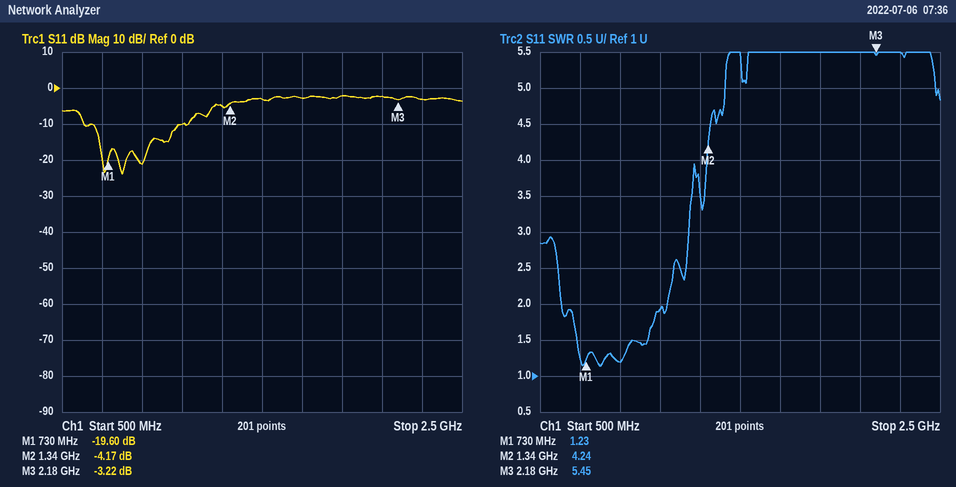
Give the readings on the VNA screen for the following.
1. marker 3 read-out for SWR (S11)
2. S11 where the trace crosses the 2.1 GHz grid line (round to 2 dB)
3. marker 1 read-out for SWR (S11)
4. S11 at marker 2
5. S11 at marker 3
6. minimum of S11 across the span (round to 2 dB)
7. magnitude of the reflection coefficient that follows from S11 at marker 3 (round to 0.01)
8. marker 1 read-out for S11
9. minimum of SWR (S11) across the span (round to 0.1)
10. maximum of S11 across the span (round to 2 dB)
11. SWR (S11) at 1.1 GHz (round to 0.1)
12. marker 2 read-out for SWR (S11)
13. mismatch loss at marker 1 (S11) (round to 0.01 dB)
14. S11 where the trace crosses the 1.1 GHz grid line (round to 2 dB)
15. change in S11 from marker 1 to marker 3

5.45
-2 dB
1.23
-4.17 dB
-3.22 dB
-24 dB
0.69
-19.60 dB
1.1
-2 dB
1.9
4.24
0.05 dB
-10 dB
16.38 dB
